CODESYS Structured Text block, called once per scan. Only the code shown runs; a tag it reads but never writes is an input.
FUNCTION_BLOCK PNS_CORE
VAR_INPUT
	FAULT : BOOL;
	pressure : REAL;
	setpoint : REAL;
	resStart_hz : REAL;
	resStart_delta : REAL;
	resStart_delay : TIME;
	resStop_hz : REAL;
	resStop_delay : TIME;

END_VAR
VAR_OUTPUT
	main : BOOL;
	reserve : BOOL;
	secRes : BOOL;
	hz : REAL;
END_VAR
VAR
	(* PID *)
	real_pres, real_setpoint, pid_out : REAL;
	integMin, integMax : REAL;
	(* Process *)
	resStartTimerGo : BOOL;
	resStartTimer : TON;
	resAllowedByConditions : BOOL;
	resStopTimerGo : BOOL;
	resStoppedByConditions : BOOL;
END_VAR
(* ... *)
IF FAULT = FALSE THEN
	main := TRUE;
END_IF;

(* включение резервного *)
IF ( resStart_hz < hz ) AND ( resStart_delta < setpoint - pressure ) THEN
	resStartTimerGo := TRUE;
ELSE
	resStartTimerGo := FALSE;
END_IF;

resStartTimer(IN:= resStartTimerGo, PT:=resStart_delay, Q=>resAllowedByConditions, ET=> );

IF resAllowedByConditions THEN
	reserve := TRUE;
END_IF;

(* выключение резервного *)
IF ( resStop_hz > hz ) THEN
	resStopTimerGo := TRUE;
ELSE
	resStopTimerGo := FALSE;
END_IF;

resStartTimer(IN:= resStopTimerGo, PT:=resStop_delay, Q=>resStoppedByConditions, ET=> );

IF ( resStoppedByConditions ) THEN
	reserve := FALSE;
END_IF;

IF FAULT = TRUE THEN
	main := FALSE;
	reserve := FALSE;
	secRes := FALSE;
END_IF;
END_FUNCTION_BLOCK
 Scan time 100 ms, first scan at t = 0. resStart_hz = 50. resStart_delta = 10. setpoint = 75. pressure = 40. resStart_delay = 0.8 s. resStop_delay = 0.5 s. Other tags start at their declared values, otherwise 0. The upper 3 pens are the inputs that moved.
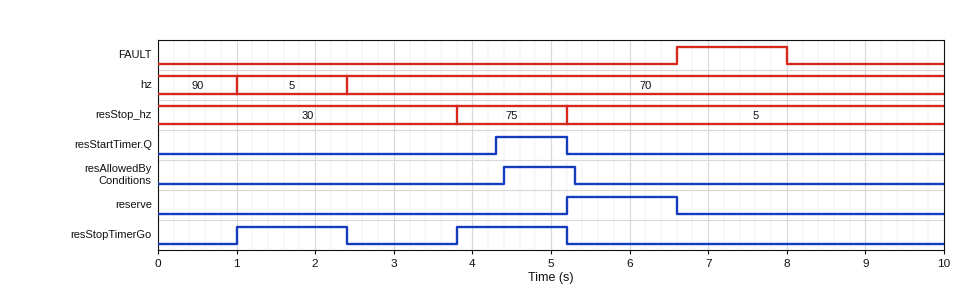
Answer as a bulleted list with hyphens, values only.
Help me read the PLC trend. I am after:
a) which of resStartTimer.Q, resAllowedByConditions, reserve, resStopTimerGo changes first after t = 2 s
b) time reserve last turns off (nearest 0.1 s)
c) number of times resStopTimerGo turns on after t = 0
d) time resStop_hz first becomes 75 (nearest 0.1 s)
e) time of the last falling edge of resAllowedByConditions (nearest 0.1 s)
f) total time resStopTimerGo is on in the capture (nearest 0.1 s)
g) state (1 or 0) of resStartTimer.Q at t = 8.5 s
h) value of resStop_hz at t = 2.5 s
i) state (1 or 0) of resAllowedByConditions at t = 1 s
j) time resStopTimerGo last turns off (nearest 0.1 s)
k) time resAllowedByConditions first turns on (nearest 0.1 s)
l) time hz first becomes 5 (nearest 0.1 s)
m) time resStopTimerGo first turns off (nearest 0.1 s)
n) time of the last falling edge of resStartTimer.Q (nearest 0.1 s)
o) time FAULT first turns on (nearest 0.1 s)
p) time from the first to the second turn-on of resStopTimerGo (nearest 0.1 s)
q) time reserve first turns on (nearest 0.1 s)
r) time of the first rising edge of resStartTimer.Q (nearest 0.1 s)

- resStopTimerGo
- 6.6 s
- 2
- 3.8 s
- 5.3 s
- 2.8 s
- 0
- 30
- 0
- 5.2 s
- 4.4 s
- 1.0 s
- 2.4 s
- 5.2 s
- 6.6 s
- 2.8 s
- 5.2 s
- 4.3 s
